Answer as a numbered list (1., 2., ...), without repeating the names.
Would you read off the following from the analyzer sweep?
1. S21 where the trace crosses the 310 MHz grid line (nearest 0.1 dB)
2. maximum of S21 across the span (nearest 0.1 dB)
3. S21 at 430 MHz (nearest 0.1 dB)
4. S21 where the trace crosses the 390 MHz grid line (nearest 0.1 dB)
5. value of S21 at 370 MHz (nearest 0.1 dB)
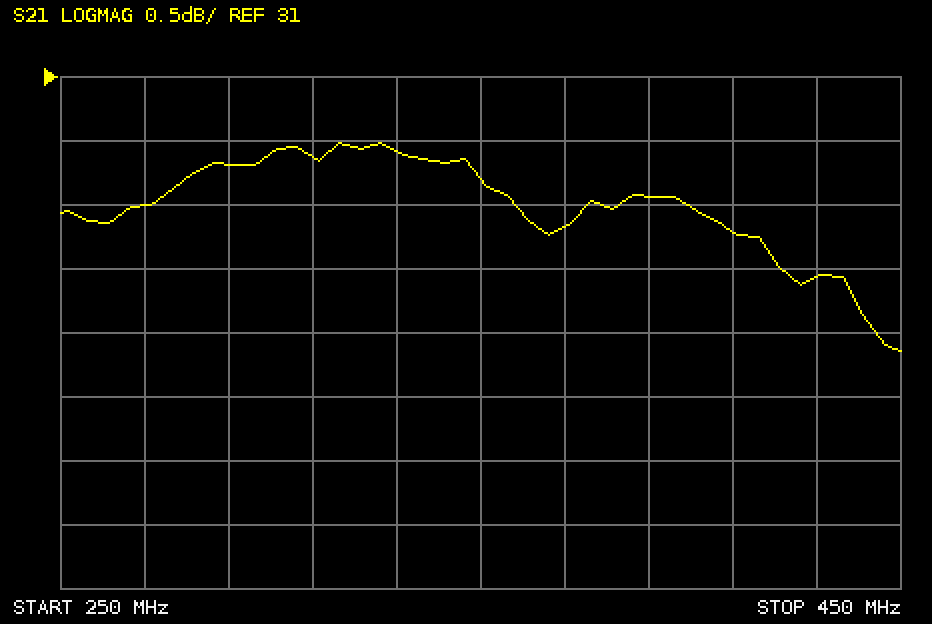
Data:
1. 30.4 dB
2. 30.5 dB
3. 29.4 dB
4. 30.1 dB
5. 29.8 dB
